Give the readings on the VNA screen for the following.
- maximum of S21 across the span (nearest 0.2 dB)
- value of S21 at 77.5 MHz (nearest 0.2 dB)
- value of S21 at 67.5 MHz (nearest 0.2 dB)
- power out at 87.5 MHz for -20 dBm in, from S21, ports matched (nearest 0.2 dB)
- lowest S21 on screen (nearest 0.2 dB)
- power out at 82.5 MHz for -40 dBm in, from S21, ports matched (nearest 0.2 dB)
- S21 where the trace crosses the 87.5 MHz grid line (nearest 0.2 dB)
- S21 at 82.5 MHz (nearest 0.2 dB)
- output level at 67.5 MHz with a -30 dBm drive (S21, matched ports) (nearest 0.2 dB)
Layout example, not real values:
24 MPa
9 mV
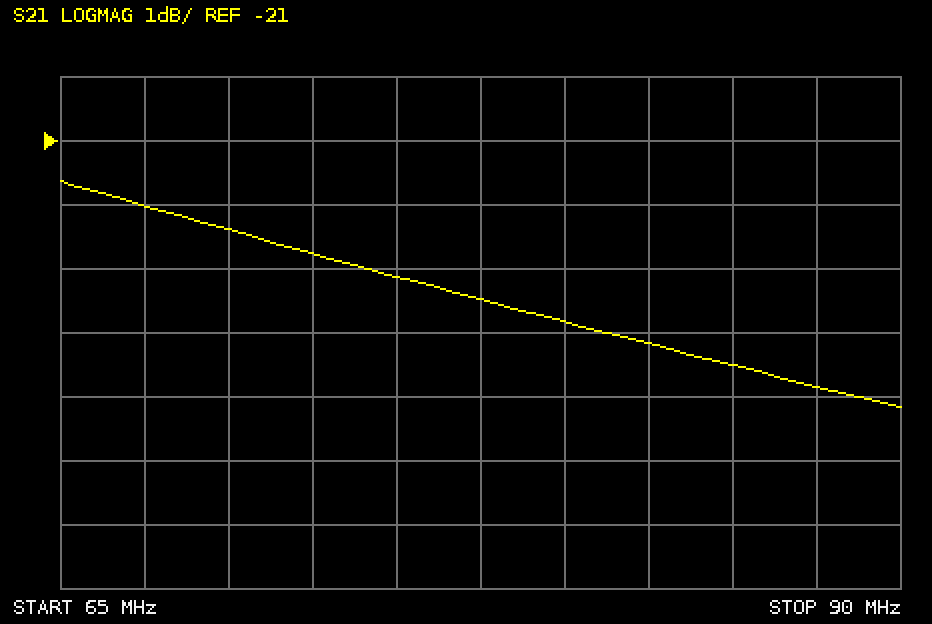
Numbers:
-21.6 dB
-23.4 dB
-22.0 dB
-44.8 dBm
-25.2 dB
-64.2 dBm
-24.8 dB
-24.2 dB
-52.0 dBm
